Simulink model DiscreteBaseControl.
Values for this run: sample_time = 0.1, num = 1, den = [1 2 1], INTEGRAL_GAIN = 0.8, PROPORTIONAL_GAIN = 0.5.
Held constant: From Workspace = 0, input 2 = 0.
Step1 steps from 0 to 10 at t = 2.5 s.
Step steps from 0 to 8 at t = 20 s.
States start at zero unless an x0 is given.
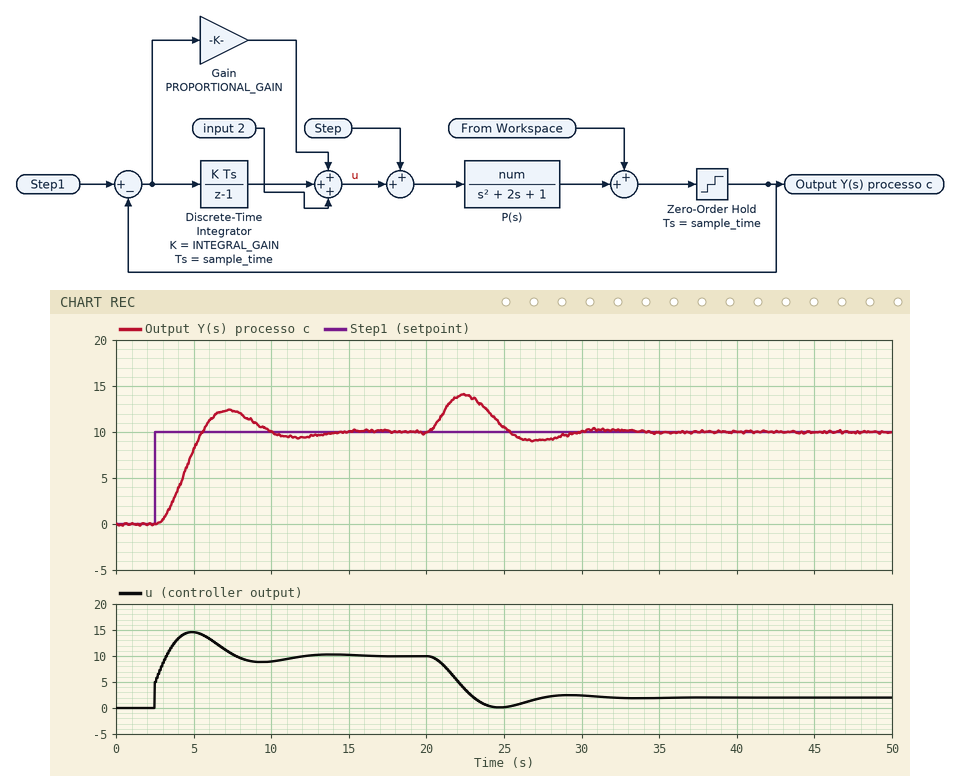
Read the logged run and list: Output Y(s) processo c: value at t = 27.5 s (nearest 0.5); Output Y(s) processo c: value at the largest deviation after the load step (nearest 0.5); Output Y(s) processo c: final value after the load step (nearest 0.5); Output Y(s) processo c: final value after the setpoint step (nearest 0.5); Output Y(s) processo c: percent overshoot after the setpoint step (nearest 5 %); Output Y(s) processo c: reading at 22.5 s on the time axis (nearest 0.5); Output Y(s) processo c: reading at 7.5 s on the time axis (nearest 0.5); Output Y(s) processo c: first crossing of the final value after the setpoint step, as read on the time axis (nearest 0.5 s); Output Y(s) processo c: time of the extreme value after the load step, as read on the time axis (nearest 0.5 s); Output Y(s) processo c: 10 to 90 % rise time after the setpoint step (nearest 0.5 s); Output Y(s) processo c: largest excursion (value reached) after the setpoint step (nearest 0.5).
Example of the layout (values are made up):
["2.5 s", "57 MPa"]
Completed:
["9.0", "14.0", "10.0", "10.0", "25 %", "14.0", "12.5", "5.5 s", "22.5 s", "2.0 s", "12.5"]
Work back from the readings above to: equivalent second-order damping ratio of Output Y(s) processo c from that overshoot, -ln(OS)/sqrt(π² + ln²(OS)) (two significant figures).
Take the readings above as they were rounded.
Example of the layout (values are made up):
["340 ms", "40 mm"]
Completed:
["0.40"]
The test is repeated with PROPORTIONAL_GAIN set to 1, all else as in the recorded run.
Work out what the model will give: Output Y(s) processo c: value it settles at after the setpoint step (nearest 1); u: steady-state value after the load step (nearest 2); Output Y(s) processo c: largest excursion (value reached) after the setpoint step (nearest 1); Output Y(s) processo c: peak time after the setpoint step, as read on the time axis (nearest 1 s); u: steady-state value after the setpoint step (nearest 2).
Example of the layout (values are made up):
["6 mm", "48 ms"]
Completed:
["10", "2", "11", "6 s", "10"]
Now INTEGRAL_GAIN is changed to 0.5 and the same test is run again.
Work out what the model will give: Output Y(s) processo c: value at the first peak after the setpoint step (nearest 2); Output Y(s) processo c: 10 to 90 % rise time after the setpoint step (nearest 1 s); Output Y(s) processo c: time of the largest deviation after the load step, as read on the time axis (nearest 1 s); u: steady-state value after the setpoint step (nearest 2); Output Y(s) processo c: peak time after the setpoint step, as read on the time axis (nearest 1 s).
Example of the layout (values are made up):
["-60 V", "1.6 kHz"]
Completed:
["10", "3 s", "23 s", "10", "9 s"]
